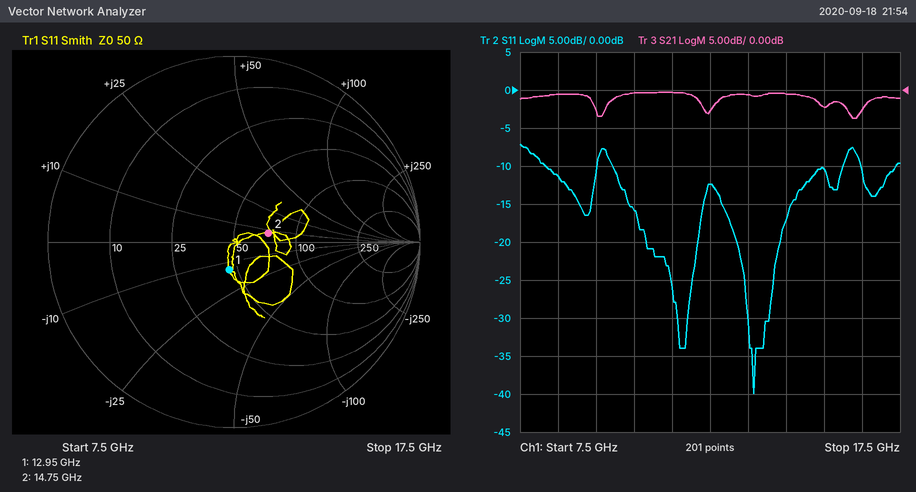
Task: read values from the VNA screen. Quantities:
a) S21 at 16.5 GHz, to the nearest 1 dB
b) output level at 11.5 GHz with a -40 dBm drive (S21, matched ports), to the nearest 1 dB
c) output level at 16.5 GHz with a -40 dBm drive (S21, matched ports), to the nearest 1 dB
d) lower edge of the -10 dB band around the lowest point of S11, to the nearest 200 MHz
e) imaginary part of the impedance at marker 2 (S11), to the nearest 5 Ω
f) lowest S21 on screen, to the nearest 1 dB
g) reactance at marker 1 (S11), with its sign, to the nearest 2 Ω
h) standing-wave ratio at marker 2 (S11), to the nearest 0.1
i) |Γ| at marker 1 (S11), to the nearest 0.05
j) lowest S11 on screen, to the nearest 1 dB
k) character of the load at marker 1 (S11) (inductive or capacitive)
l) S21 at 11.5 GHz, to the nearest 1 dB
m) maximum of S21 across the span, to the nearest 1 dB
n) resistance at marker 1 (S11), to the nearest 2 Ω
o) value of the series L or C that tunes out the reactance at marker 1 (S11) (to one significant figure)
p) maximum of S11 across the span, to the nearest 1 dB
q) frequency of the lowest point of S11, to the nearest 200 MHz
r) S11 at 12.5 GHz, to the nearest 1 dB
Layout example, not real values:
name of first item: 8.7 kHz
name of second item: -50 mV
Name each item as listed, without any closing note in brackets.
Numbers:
S21 at 16.5 GHz, to the nearest 1 dB: -3 dB
output level at 11.5 GHz with a -40 dBm drive (S21, matched ports), to the nearest 1 dB: -40 dBm
output level at 16.5 GHz with a -40 dBm drive (S21, matched ports), to the nearest 1 dB: -43 dBm
lower edge of the -10 dB band around the lowest point of S11, to the nearest 200 MHz: 10.0 GHz
imaginary part of the impedance at marker 2 (S11), to the nearest 5 Ω: +5 Ω
lowest S21 on screen, to the nearest 1 dB: -4 dB
reactance at marker 1 (S11), with its sign, to the nearest 2 Ω: -14 Ω
standing-wave ratio at marker 2 (S11), to the nearest 0.1: 1.5
|Γ| at marker 1 (S11), to the nearest 0.05: 0.15
lowest S11 on screen, to the nearest 1 dB: -40 dB
character of the load at marker 1 (S11): capacitive
S21 at 11.5 GHz, to the nearest 1 dB: 0 dB
maximum of S21 across the span, to the nearest 1 dB: 0 dB
resistance at marker 1 (S11), to the nearest 2 Ω: 46 Ω
value of the series L or C that tunes out the reactance at marker 1 (S11): 200 pH
maximum of S11 across the span, to the nearest 1 dB: -7 dB
frequency of the lowest point of S11, to the nearest 200 MHz: 13.6 GHz
S11 at 12.5 GHz, to the nearest 1 dB: -12 dB
